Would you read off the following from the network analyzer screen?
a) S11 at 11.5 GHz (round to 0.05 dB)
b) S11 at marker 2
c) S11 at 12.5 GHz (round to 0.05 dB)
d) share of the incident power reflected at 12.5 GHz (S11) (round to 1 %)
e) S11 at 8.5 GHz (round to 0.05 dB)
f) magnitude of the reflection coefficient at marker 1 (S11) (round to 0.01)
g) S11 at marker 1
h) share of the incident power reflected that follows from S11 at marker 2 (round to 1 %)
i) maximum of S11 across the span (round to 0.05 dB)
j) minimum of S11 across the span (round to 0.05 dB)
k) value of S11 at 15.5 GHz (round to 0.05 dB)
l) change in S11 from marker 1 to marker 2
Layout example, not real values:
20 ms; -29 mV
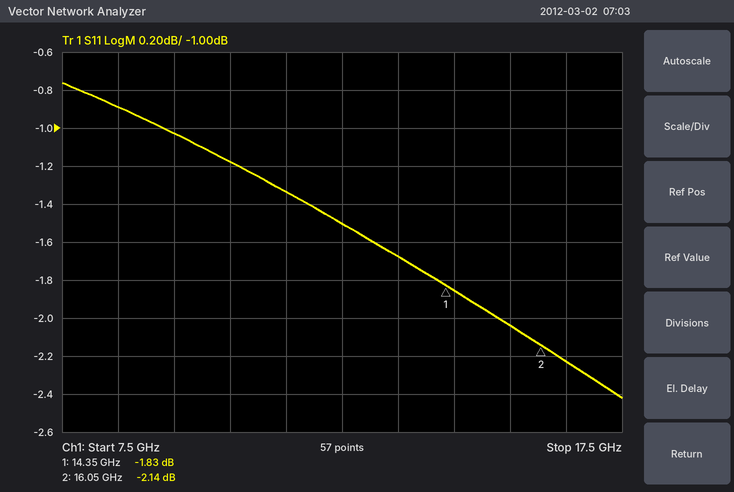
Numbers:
-1.35 dB; -2.14 dB; -1.50 dB; 71 %; -0.90 dB; 0.81; -1.83 dB; 61 %; -0.75 dB; -2.40 dB; -2.05 dB; -0.31 dB
